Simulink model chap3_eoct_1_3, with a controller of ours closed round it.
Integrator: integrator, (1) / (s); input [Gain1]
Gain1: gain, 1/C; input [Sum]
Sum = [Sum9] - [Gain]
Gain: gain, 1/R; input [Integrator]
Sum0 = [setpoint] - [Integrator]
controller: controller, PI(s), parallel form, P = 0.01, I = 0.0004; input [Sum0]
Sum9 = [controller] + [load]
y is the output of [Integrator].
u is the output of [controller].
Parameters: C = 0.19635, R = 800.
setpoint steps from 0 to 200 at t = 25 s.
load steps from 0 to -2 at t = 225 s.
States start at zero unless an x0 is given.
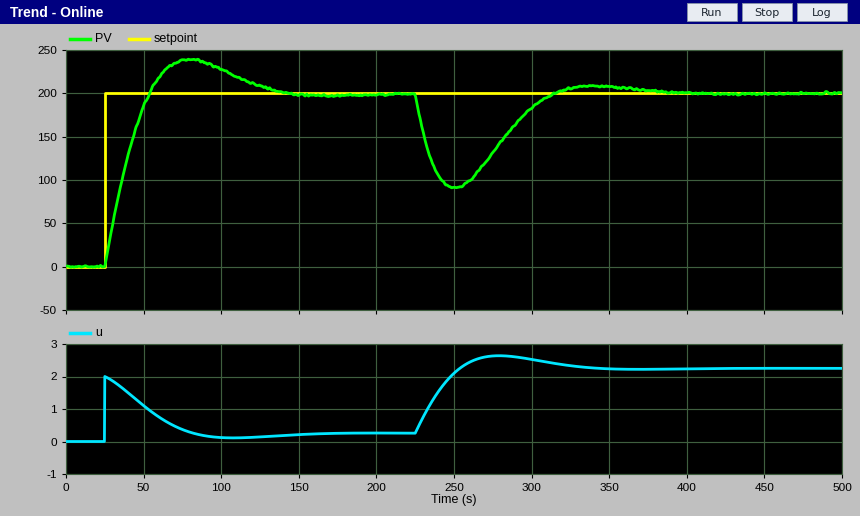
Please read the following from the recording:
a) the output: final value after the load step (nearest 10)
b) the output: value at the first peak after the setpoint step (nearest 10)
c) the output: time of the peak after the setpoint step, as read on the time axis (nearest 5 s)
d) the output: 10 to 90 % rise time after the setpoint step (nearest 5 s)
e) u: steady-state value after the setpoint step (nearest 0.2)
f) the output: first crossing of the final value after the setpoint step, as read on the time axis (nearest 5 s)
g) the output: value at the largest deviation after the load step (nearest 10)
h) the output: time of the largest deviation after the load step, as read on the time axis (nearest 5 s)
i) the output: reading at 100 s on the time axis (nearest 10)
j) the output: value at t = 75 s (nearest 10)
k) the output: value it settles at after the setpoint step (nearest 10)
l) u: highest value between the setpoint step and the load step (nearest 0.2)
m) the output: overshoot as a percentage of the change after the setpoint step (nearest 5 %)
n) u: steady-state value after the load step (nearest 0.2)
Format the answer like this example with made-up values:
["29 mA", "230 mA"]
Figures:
["200", "240", "80 s", "20 s", "0.2", "55 s", "90", "250 s", "230", "240", "200", "2.0", "20 %", "2.2"]
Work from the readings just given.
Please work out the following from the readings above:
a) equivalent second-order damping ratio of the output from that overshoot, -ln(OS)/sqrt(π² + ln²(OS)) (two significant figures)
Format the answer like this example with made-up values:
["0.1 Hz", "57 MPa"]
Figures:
["0.46"]
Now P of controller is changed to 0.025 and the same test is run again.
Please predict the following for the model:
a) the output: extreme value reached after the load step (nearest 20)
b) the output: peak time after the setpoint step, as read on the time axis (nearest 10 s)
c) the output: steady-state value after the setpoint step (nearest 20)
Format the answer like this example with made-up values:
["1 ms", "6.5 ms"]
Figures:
["140", "70 s", "200"]
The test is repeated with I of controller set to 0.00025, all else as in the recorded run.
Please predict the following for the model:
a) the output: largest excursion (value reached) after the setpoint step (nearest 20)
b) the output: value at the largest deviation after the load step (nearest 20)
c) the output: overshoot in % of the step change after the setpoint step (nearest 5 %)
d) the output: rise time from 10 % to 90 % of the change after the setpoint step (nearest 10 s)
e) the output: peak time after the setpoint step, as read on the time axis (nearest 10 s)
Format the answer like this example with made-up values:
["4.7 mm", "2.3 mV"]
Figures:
["220", "80", "15 %", "30 s", "90 s"]
